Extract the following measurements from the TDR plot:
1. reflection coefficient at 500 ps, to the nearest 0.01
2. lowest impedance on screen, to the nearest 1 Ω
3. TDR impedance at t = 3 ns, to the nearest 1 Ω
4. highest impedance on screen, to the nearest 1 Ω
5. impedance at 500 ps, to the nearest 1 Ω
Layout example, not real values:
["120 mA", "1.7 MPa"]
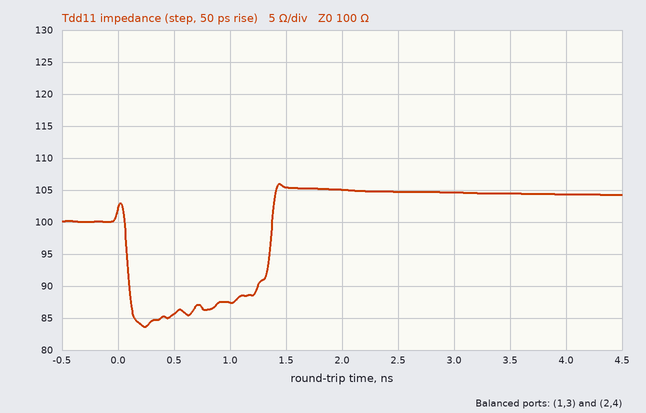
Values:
["-0.08", "84 Ω", "105 Ω", "106 Ω", "86 Ω"]
